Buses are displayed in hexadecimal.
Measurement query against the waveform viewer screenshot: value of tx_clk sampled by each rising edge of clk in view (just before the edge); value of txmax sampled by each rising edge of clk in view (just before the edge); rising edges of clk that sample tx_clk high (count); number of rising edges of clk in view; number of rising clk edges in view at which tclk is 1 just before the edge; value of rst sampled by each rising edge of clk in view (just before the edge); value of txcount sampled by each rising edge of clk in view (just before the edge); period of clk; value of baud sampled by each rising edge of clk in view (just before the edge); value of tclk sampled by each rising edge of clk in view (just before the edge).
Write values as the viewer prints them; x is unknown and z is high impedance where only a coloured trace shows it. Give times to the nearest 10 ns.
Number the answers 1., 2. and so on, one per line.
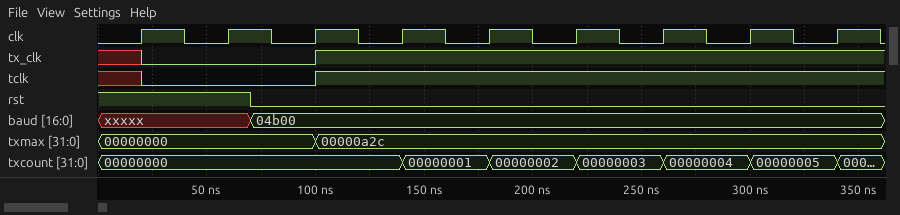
1. x 0 0 1 1 1 1 1 1
2. 00000000, 00000000, 00000000, 00000a2c, 00000a2c, 00000a2c, 00000a2c, 00000a2c, 00000a2c
3. 6
4. 9
5. 6
6. 1 1 0 0 0 0 0 0 0
7. 00000000, 00000000, 00000000, 00000000, 00000001, 00000002, 00000003, 00000004, 00000005
8. 40 ns
9. xxxxx, xxxxx, 04b00, 04b00, 04b00, 04b00, 04b00, 04b00, 04b00
10. x 0 0 1 1 1 1 1 1
